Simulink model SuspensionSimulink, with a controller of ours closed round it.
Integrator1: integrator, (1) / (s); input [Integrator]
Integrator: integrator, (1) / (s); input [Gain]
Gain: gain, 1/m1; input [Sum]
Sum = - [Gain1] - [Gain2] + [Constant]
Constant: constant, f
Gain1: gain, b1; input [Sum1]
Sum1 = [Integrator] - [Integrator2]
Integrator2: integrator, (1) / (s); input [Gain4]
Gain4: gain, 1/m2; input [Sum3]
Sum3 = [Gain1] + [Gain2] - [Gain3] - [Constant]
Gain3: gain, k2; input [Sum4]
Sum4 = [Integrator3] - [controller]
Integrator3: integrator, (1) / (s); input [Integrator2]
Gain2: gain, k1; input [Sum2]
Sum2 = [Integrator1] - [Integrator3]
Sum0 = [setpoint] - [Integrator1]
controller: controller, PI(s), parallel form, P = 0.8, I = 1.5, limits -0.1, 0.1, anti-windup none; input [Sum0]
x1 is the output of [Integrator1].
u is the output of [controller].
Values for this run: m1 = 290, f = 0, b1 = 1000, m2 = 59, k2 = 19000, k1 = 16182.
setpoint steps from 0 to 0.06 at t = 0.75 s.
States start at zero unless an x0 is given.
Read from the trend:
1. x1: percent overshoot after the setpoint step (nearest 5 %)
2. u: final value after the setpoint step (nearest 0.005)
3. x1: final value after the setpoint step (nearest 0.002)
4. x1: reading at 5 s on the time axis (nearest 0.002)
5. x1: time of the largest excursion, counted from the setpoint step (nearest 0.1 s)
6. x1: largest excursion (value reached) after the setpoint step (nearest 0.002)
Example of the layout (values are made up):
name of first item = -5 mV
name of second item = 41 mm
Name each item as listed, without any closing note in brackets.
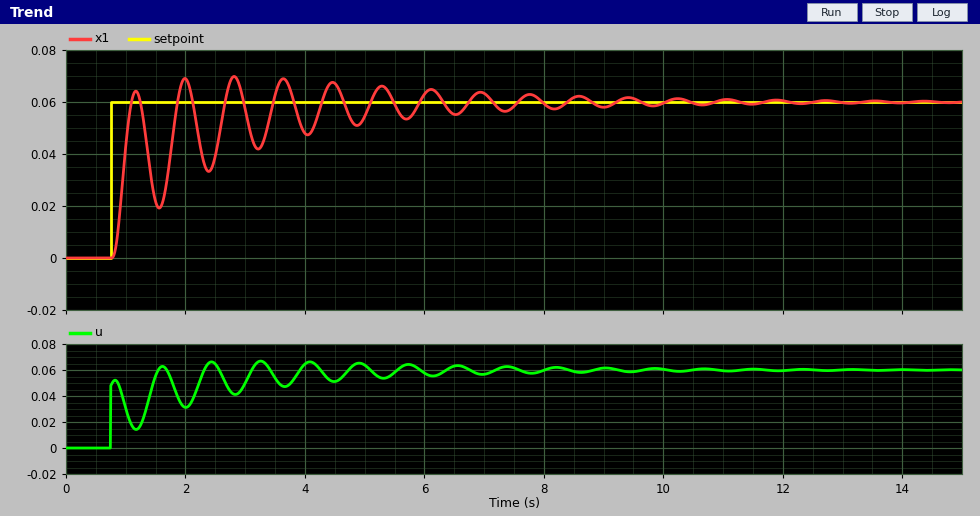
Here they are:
x1: percent overshoot after the setpoint step = 15 %
u: final value after the setpoint step = 0.060
x1: final value after the setpoint step = 0.060
x1: reading at 5 s on the time axis = 0.054
x1: time of the largest excursion, counted from the setpoint step = 2.1 s
x1: largest excursion (value reached) after the setpoint step = 0.070
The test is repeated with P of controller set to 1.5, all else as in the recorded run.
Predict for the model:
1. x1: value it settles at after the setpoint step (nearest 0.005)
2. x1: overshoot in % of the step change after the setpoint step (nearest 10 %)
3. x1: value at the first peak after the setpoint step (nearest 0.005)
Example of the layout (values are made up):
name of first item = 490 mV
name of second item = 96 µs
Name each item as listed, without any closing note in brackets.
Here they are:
x1: value it settles at after the setpoint step = 0.060
x1: overshoot in % of the step change after the setpoint step = 30 %
x1: value at the first peak after the setpoint step = 0.075
